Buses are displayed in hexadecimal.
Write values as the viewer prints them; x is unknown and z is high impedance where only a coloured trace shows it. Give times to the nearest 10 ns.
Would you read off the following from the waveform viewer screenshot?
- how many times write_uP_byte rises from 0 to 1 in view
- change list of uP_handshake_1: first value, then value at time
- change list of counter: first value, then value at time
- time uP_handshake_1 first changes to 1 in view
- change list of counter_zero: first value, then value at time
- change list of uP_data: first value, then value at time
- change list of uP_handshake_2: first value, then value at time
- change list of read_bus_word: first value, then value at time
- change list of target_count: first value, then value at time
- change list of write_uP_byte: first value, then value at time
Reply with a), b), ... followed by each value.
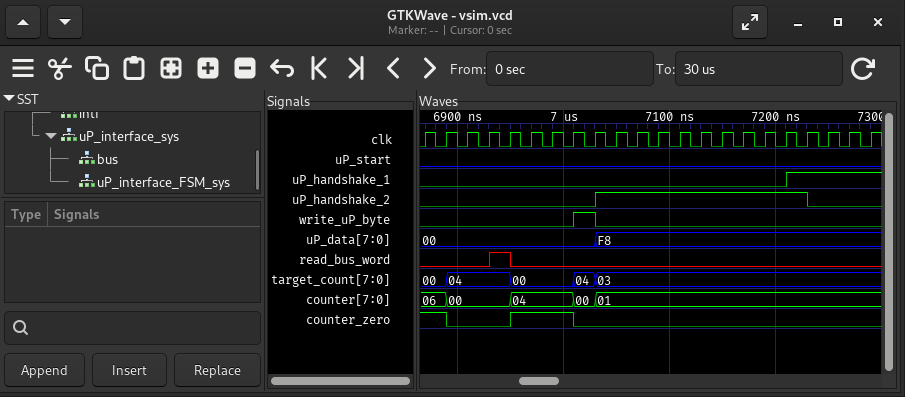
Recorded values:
a) 1
b) 0, 1 at 7210 ns
c) 06, 00 at 6890 ns, 04 at 6950 ns, 00 at 7010 ns, 01 at 7030 ns
d) 7210 ns
e) 1, 0 at 6890 ns, 1 at 6950 ns, 0 at 7010 ns
f) 00, F8 at 7030 ns
g) 0, 1 at 7030 ns, 0 at 7230 ns
h) 0, 1 at 6930 ns, 0 at 6950 ns
i) 00, 04 at 6890 ns, 00 at 6950 ns, 04 at 7010 ns, 03 at 7030 ns
j) 0, 1 at 7010 ns, 0 at 7030 ns
